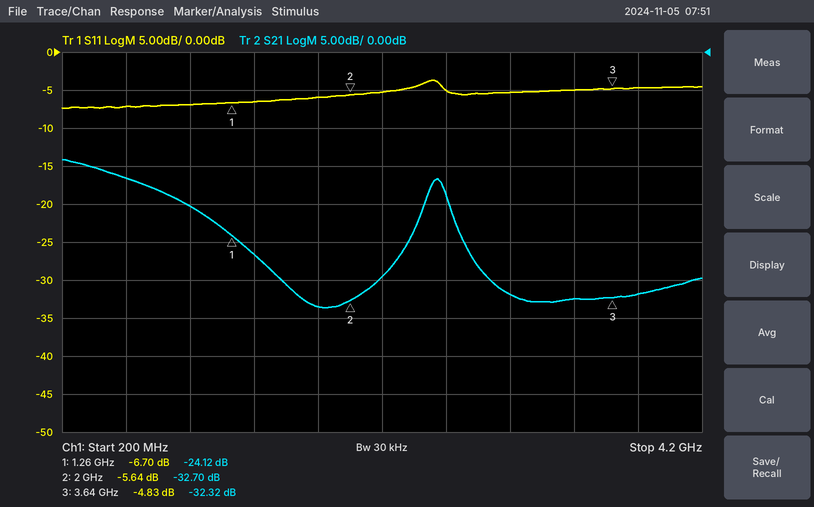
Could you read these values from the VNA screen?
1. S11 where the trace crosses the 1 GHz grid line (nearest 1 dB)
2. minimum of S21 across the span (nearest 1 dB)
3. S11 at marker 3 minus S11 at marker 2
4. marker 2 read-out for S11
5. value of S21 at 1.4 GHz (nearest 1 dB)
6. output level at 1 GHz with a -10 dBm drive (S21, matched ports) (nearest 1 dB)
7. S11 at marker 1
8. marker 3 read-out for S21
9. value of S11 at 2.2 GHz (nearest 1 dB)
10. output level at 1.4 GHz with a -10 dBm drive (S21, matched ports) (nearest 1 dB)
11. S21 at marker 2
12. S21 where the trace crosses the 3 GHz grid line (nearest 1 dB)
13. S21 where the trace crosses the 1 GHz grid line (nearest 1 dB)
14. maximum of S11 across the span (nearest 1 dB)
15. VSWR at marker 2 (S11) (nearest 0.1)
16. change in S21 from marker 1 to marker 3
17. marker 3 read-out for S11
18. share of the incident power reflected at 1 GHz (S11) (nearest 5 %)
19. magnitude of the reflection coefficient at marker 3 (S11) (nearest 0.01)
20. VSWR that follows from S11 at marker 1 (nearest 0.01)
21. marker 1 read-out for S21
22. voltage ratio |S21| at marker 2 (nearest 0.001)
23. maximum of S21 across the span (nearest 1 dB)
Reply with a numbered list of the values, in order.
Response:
1. -7 dB
2. -34 dB
3. 0.81 dB
4. -5.64 dB
5. -27 dB
6. -30 dBm
7. -6.70 dB
8. -32.32 dB
9. -5 dB
10. -37 dBm
11. -32.70 dB
12. -32 dB
13. -20 dB
14. -4 dB
15. 3.2
16. -8.20 dB
17. -4.83 dB
18. 20 %
19. 0.57
20. 2.72
21. -24.12 dB
22. 0.023
23. -14 dB
